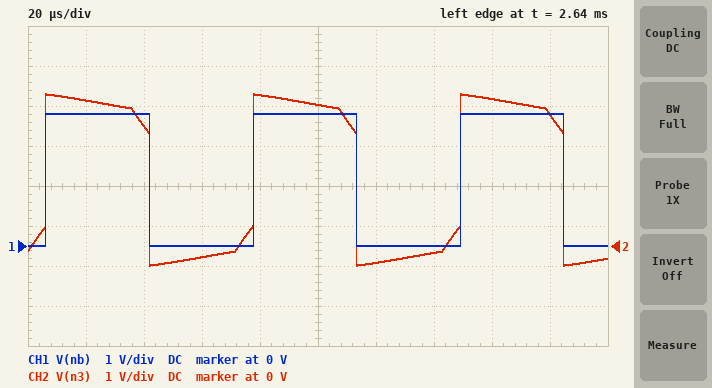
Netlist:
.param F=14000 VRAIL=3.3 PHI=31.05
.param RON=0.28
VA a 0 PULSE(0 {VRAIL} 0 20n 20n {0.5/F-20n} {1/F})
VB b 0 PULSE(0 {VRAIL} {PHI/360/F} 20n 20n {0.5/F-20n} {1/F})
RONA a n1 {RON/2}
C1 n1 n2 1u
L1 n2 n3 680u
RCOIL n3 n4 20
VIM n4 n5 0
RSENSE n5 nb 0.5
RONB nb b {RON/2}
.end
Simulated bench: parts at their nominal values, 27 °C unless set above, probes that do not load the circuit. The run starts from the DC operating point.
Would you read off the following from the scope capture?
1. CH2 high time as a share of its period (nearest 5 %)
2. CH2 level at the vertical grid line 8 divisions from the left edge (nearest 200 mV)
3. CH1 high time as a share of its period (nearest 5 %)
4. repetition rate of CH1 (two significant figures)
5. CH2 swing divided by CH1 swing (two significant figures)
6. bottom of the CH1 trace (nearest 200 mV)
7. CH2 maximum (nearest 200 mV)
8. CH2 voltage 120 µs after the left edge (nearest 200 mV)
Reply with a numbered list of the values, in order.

1. 50 %
2. 3.6 V
3. 50 %
4. 14 kHz
5. 1.3
6. 0 V
7. 3.8 V
8. -400 mV
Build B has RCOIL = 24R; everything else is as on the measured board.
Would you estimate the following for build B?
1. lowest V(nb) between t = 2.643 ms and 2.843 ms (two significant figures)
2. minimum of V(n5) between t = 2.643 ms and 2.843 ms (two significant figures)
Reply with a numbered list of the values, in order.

1. -3.4 mV
2. -16 mV
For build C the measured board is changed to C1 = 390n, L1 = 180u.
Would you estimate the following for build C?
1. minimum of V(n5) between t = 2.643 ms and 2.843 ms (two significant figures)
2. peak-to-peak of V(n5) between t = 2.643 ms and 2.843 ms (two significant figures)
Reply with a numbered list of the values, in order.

1. -48 mV
2. 3.4 V
